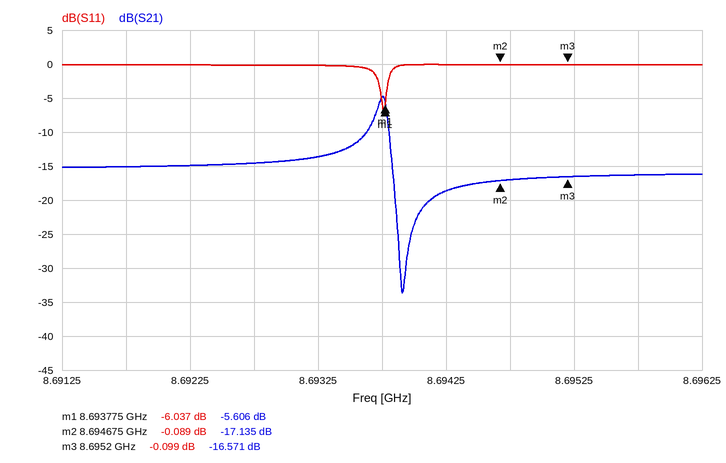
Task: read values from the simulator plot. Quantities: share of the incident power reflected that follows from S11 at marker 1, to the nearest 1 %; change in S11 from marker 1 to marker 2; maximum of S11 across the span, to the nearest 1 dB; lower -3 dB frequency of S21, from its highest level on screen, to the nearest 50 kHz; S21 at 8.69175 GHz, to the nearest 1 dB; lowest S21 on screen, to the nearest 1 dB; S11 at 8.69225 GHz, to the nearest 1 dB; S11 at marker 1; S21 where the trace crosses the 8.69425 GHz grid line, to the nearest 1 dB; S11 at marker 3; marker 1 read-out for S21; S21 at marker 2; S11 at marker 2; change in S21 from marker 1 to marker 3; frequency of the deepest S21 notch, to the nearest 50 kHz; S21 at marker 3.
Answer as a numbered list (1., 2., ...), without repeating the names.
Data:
1. 25 %
2. 5.948 dB
3. 0 dB
4. 8.69370 GHz
5. -15 dB
6. -34 dB
7. 0 dB
8. -6.037 dB
9. -19 dB
10. -0.099 dB
11. -5.606 dB
12. -17.135 dB
13. -0.089 dB
14. -10.965 dB
15. 8.69390 GHz
16. -16.571 dB
